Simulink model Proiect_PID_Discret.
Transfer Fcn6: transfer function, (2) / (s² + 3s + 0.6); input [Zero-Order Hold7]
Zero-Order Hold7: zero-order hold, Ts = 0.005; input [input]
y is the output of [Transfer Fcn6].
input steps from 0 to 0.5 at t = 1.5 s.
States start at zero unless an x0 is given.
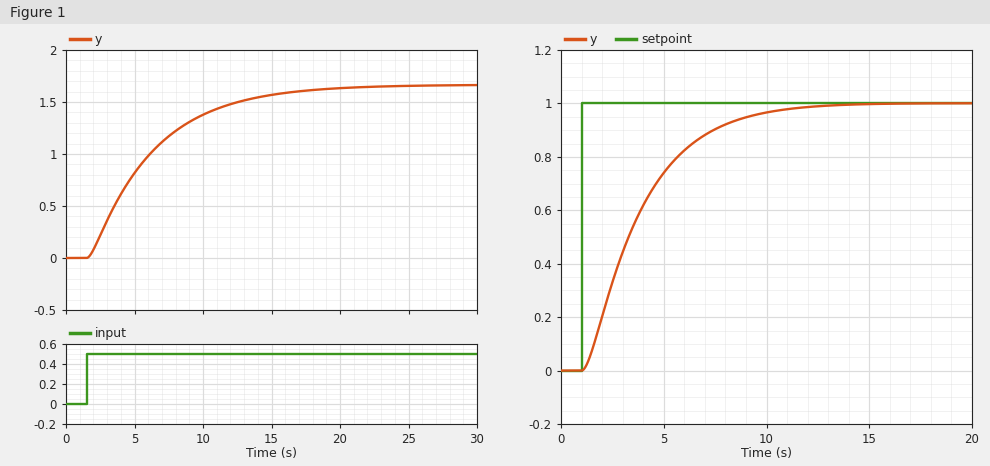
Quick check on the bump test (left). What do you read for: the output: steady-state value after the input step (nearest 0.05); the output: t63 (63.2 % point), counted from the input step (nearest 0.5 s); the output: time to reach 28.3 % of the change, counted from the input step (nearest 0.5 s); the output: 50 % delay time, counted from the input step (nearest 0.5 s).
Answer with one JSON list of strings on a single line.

["1.65", "5.0 s", "2.0 s", "3.5 s"]
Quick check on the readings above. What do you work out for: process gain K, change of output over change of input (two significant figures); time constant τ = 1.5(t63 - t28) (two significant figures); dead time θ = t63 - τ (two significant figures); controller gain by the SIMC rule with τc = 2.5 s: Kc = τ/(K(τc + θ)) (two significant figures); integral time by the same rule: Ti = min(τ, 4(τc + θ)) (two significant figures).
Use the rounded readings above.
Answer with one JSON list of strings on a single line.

["3.3", "4.5 s", "0.50 s", "0.45", "4.5 s"]
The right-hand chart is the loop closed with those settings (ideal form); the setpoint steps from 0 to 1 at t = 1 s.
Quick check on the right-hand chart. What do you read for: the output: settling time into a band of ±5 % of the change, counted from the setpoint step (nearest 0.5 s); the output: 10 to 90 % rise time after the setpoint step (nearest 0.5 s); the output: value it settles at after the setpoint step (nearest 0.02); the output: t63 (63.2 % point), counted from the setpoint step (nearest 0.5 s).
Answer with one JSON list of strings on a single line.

["8.0 s", "6.0 s", "1.00", "3.0 s"]
